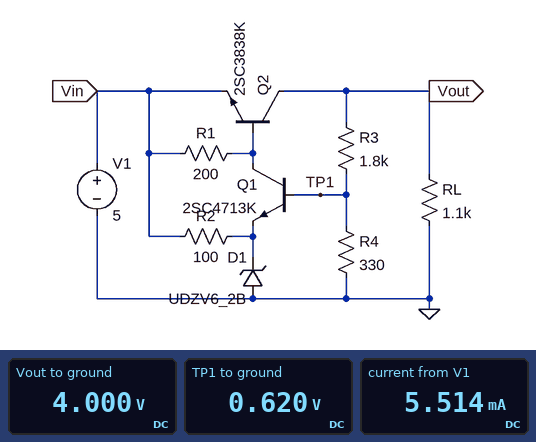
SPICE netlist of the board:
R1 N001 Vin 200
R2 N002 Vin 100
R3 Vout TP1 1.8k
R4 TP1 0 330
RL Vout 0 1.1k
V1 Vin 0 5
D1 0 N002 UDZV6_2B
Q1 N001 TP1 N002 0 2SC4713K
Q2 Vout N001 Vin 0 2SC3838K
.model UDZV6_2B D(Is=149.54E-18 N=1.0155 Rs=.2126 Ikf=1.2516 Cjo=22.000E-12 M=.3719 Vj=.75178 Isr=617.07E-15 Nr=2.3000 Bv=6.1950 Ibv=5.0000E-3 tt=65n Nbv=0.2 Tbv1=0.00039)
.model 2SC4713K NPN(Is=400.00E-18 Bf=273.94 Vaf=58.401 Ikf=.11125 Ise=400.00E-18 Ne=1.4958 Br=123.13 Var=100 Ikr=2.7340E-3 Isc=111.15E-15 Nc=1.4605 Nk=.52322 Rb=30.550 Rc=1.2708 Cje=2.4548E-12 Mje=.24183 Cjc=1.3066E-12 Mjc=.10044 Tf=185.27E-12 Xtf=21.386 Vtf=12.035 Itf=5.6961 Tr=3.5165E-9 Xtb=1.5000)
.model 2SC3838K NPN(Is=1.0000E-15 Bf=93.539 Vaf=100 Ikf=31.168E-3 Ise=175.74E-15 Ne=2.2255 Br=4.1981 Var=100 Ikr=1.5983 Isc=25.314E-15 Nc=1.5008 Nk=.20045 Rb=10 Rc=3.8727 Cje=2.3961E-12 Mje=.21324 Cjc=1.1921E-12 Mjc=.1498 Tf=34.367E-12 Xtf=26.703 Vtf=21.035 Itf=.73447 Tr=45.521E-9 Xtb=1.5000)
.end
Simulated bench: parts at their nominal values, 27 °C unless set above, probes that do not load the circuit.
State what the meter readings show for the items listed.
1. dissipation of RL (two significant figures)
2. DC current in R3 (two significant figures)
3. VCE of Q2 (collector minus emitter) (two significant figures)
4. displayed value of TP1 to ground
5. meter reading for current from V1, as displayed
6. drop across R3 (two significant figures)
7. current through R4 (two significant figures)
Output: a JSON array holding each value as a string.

["15 mW", "1.9 mA", "-1.0 V", "0.620 V", "5.514 mA", "3.4 V", "1.9 mA"]
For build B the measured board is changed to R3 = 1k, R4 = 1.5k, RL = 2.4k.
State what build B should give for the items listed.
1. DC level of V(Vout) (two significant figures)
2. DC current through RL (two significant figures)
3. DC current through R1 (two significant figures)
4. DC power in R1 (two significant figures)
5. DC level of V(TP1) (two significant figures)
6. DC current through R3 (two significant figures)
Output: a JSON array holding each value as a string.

["4.1 V", "1.7 mA", "650 µA", "85 µW", "2.5 V", "1.6 mA"]
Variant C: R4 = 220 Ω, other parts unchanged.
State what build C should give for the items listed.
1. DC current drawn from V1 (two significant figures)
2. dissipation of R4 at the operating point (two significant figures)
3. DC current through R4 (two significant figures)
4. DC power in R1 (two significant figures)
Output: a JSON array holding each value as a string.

["5.6 mA", "860 µW", "2.0 mA", "240 µW"]
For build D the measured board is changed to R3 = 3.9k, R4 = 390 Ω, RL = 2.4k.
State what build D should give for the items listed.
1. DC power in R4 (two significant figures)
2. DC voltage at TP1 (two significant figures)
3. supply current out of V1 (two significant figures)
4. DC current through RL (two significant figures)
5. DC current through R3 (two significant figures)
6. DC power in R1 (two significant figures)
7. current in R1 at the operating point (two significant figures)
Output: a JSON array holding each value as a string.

["360 µW", "380 mV", "2.7 mA", "1.7 mA", "970 µA", "55 µW", "520 µA"]
